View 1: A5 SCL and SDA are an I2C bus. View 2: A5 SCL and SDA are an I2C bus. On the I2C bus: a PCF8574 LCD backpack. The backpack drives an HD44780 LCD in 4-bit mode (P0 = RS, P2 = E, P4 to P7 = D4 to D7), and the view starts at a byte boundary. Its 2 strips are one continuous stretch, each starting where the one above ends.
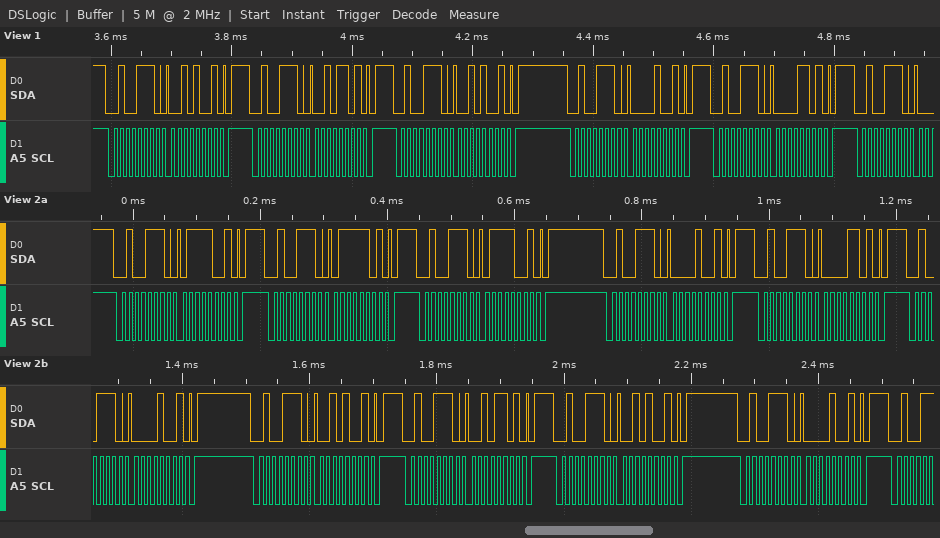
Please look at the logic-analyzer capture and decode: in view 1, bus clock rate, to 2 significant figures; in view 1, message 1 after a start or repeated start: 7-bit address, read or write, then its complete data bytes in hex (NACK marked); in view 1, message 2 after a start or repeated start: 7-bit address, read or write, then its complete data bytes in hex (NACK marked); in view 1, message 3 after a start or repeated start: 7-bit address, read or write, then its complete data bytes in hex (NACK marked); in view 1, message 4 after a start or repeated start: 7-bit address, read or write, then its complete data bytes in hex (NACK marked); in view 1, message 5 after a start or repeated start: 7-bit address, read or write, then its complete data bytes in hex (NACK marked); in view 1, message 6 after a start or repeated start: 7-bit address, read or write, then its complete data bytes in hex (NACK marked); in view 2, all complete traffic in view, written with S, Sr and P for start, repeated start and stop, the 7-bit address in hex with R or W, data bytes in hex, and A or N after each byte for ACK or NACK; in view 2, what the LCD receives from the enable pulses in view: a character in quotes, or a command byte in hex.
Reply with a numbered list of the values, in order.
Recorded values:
1. 100 kHz
2. 0x27 write: 29
3. 0x27 write: 2D
4. 0x27 write: 29
5. 0x27 write: 09
6. 0x27 write: 0D
7. 0x27 write
8. S 27W A 79 A P S 27W A 7D A P S 27W A 79 A P S 27W A 09 A P S 27W A 0D A P S 27W A 09 A P S 27W A 29 A P S 27W A 2D A P S 27W A 29 A P S 27W A 09 A P
9. 'p'
